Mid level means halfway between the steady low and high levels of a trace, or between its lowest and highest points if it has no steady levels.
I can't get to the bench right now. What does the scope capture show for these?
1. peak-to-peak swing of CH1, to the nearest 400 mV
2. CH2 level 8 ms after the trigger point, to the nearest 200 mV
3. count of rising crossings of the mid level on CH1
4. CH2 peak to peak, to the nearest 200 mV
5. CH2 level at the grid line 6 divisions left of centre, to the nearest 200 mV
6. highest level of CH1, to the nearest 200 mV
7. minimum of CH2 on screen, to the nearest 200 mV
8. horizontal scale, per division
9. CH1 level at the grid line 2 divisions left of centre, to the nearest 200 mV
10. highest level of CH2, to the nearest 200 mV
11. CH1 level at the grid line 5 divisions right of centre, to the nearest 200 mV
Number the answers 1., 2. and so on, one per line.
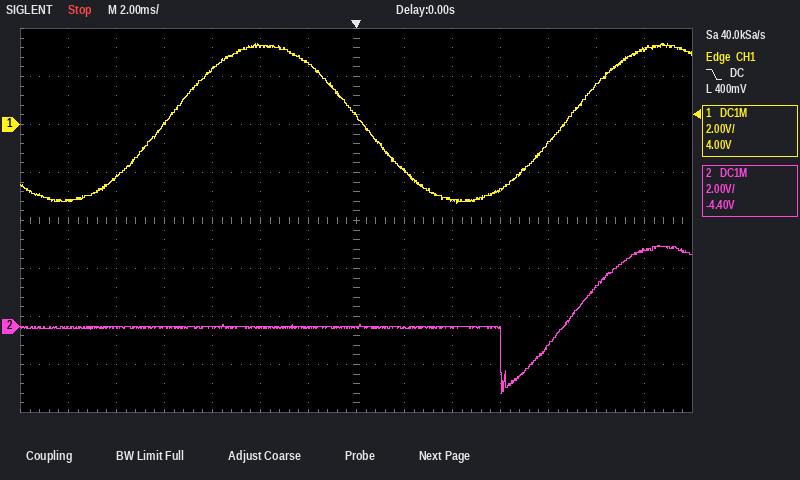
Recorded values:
1. 6.8 V
2. -800 mV
3. 2
4. 6.2 V
5. 0.0 V
6. 3.4 V
7. -2.8 V
8. 2 ms
9. 3.2 V
10. 3.4 V
11. 1.6 V
